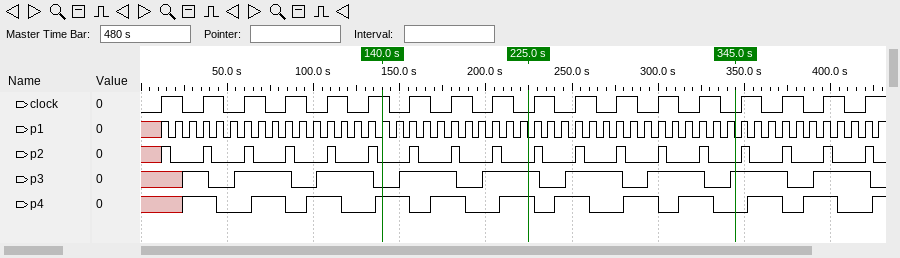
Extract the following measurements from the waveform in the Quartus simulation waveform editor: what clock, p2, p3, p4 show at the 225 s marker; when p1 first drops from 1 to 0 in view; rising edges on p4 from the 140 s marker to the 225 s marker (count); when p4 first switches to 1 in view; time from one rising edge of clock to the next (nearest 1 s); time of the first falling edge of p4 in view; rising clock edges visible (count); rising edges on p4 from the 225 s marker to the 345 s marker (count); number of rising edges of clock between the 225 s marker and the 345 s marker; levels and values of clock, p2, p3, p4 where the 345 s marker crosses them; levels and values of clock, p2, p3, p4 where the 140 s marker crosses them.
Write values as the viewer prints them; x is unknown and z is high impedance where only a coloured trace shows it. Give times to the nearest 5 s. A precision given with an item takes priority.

clock=0, p2=0, p3=1, p4=1
15 s
2
25 s
24 s
45 s
18
3
5
clock=0, p2=0, p3=1, p4=0
clock=1, p2=0, p3=0, p4=1
